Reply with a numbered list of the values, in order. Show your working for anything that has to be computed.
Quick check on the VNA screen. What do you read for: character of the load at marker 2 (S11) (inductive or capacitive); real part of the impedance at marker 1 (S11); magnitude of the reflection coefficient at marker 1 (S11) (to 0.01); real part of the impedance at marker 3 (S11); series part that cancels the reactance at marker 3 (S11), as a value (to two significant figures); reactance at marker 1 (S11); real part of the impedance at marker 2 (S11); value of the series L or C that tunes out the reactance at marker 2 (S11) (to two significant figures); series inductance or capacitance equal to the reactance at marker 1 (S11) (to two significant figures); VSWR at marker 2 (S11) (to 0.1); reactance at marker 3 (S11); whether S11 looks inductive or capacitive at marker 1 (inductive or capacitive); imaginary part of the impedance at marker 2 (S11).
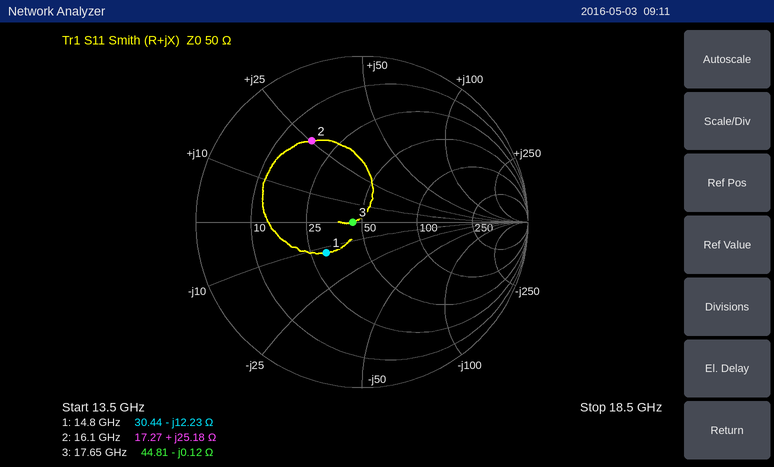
1. inductive
2. 30.44 Ω
3. 0.28
4. 44.81 Ω
5. L = 0.12 Ω/(2π × 17.65 GHz) ≈ 1.1 pH
6. -12.23 Ω
7. 17.27 Ω
8. C = 1/(2π × 16.1 GHz × 25.18 Ω) ≈ 393 fF, so 390 fF to two significant figures
9. C = 1/(2π × 14.8 GHz × 12.23 Ω) ≈ 879 fF, so 880 fF to two significant figures
10. 3.7
11. -0.12 Ω
12. capacitive
13. +25.18 Ω
